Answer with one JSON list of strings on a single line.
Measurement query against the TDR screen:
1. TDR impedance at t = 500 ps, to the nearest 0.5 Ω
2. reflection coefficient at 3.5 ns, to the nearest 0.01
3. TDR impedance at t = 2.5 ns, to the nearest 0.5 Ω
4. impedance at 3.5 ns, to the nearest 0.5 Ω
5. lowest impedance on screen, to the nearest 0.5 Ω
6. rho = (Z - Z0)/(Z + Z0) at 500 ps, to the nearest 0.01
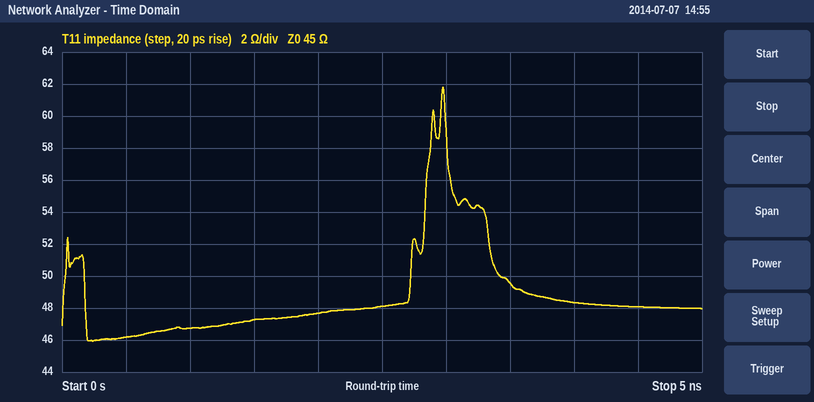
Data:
["46.0 Ω", "+0.05", "48.0 Ω", "49.5 Ω", "46.0 Ω", "+0.01"]
